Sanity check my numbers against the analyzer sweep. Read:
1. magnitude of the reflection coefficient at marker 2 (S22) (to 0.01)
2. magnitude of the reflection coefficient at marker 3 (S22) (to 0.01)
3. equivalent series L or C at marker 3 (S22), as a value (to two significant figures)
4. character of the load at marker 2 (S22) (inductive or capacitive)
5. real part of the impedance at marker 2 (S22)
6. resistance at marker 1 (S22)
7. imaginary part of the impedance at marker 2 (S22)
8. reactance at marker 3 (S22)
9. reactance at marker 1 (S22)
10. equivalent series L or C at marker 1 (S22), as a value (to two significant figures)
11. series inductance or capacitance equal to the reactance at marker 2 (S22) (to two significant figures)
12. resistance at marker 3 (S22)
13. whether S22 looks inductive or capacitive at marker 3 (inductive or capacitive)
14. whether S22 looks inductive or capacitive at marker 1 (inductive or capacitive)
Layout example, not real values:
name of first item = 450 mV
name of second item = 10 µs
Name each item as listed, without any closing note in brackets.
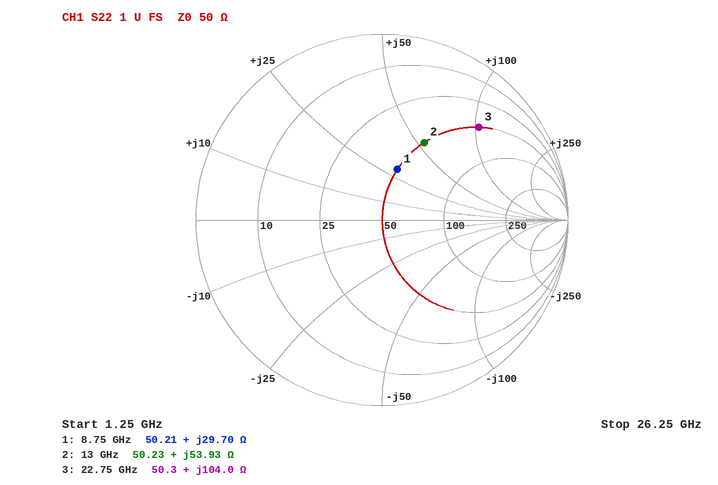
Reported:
magnitude of the reflection coefficient at marker 2 (S22) = 0.47
magnitude of the reflection coefficient at marker 3 (S22) = 0.72
equivalent series L or C at marker 3 (S22), as a value = 730 pH
character of the load at marker 2 (S22) = inductive
real part of the impedance at marker 2 = 50.23 Ω
resistance at marker 1 = 50.21 Ω
imaginary part of the impedance at marker 2 = +53.93 Ω
reactance at marker 3 = +104.0 Ω
reactance at marker 1 = +29.70 Ω
equivalent series L or C at marker 1 (S22), as a value = 540 pH
series inductance or capacitance equal to the reactance at marker 2 (S22) = 660 pH
resistance at marker 3 = 50.3 Ω
whether S22 looks inductive or capacitive at marker 3 = inductive
whether S22 looks inductive or capacitive at marker 1 = inductive
